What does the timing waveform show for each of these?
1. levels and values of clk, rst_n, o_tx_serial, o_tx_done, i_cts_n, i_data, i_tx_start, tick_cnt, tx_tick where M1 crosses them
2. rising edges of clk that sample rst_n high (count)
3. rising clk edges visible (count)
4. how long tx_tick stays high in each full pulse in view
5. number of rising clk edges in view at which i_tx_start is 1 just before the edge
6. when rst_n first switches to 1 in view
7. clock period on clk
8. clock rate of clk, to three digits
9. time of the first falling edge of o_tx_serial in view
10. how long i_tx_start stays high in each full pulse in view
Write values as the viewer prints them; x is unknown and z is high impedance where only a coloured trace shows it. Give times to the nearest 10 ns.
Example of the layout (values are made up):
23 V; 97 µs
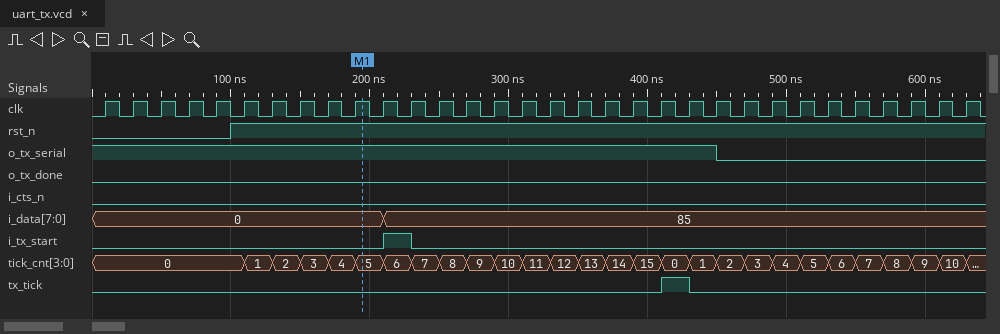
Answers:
clk=1, rst_n=1, o_tx_serial=1, o_tx_done=0, i_cts_n=0, i_data=0, i_tx_start=0, tick_cnt=5, tx_tick=0; 27; 32; 20 ns; 1; 100 ns; 20 ns; 50.0 MHz; 450 ns; 20 ns
